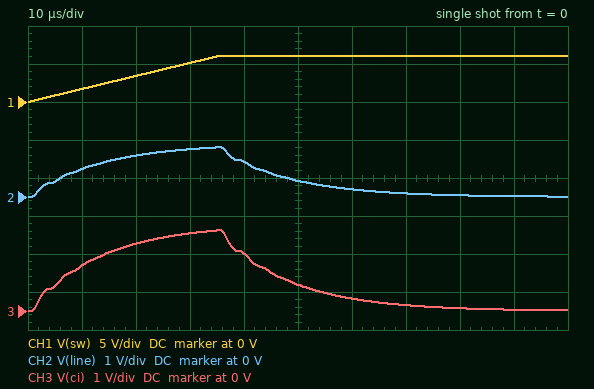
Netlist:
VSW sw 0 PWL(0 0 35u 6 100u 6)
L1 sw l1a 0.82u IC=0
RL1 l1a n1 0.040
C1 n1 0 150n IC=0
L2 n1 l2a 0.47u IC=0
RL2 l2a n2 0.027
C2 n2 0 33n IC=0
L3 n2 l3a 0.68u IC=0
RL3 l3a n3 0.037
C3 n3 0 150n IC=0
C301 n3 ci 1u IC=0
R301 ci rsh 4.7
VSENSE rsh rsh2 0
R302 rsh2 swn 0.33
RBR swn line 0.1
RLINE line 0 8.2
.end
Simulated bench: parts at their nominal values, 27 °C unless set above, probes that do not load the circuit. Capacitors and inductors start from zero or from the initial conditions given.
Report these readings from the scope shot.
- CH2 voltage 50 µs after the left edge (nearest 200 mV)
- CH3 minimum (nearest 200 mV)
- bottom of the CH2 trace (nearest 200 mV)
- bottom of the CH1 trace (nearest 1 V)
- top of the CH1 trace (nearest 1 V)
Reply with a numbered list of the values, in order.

1. 400 mV
2. 0 V
3. 0 V
4. 0 V
5. 6 V
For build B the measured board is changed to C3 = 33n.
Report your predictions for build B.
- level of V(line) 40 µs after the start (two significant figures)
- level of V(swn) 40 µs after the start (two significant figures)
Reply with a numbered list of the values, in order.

1. 890 mV
2. 900 mV
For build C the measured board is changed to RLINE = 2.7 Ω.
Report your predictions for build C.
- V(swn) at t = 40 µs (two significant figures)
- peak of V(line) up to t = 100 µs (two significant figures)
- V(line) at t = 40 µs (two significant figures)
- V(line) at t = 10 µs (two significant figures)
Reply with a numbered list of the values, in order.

1. 260 mV
2. 460 mV
3. 250 mV
4. 330 mV
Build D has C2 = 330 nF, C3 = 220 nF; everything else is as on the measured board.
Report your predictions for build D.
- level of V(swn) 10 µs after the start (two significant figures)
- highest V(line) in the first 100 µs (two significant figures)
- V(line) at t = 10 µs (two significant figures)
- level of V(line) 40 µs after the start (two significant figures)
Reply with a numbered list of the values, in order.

1. 790 mV
2. 1.3 V
3. 780 mV
4. 850 mV
